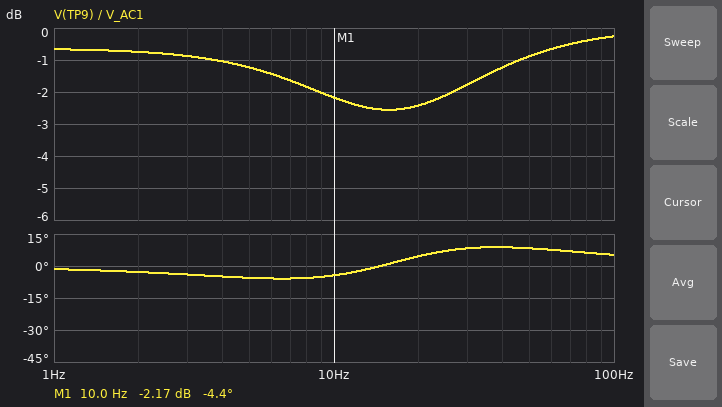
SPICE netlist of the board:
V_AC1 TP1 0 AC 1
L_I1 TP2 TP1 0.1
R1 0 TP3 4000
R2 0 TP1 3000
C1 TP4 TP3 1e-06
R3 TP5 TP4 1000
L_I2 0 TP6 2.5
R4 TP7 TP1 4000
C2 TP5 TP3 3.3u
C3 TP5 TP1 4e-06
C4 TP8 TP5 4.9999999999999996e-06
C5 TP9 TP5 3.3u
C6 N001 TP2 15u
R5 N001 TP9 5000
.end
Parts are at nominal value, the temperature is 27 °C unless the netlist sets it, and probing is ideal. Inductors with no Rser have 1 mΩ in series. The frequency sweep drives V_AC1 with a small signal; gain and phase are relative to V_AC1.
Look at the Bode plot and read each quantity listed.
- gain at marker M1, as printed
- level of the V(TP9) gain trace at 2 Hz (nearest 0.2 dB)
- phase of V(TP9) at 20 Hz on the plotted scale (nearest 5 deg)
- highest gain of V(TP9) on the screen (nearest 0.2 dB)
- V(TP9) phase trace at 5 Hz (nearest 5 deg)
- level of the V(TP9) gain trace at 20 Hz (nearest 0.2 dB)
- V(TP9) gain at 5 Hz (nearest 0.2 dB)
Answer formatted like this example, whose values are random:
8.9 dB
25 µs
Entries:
-2.17 dB
-0.8 dB
5 deg
-0.2 dB
-5 deg
-2.4 dB
-1.2 dB
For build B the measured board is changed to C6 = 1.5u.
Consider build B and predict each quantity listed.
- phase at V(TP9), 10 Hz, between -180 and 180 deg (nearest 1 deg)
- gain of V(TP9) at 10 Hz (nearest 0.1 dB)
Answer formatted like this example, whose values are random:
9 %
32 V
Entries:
8 deg
-2.6 dB
